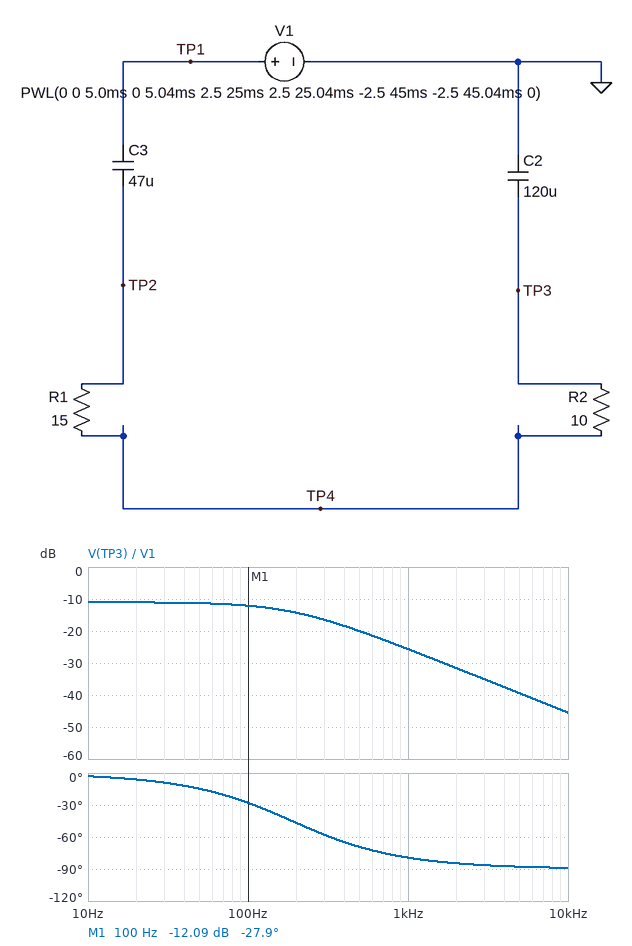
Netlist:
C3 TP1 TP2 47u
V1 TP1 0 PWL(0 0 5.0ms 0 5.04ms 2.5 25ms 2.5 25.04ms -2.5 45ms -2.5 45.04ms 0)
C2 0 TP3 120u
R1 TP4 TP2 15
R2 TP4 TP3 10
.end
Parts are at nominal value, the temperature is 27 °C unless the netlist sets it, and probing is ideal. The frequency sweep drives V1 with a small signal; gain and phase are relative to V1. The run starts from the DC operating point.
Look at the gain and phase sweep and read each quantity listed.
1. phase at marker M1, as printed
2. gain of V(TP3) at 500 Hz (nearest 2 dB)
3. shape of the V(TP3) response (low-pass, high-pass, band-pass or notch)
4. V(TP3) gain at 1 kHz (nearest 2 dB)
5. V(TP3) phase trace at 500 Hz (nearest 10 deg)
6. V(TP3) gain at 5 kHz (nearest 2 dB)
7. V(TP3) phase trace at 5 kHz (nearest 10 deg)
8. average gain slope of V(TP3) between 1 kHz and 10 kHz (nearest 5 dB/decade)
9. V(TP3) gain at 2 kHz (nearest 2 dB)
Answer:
-27.9 deg
-20 dB
low-pass
-26 dB
-70 deg
-40 dB
-90 deg
-20 dB/decade
-32 dB
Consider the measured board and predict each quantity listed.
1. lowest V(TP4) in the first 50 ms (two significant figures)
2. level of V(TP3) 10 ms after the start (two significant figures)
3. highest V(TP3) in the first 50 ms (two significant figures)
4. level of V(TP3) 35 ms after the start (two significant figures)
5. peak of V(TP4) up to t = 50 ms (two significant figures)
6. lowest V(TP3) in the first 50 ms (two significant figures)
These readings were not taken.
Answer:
-1.3 V
700 mV
700 mV
-700 mV
990 mV
-700 mV
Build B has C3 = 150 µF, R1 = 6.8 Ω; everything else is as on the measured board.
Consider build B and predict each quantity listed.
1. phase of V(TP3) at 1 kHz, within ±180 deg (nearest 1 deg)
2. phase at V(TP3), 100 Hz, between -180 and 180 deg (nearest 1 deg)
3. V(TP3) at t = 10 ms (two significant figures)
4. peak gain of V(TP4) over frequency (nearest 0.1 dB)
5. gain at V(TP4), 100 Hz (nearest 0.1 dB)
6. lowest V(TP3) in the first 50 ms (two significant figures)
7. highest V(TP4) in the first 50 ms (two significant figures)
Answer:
-82 deg
-35 deg
1.4 V
-4.5 dB
-4.9 dB
-1.4 V
1.5 V
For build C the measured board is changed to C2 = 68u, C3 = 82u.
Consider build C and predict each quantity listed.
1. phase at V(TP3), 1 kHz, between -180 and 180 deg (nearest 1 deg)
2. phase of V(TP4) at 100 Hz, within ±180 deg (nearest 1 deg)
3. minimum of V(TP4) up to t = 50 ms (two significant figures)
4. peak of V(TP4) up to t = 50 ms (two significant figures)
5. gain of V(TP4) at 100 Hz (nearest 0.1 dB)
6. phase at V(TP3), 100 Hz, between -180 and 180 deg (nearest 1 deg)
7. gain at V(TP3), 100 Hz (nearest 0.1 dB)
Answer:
-80 deg
-7 deg
-1.4 V
1.4 V
-5.8 dB
-30 deg
-6.5 dB
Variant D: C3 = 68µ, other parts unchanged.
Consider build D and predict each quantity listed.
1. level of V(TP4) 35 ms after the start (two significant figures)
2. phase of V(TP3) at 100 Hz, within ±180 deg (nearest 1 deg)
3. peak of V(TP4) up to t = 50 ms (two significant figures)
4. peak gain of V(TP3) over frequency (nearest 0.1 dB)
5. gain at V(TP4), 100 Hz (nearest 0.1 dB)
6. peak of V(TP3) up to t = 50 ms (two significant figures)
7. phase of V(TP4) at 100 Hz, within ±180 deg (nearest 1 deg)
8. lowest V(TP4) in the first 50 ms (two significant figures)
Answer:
-900 mV
-34 deg
1.0 V
-8.8 dB
-8.5 dB
900 mV
3 deg
-1.1 V
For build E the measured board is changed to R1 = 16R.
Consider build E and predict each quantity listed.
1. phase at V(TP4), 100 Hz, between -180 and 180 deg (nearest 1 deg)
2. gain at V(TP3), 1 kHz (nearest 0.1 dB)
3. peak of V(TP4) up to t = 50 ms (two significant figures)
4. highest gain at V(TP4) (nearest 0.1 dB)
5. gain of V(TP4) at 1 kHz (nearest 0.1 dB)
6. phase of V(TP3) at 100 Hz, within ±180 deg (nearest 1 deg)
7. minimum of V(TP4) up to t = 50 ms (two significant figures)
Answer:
8 deg
-26.0 dB
960 mV
-8.3 dB
-8.4 dB
-29 deg
-1.2 V
